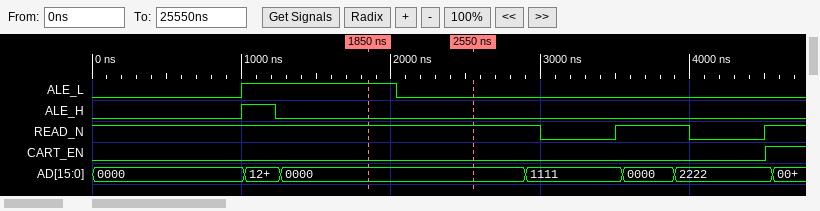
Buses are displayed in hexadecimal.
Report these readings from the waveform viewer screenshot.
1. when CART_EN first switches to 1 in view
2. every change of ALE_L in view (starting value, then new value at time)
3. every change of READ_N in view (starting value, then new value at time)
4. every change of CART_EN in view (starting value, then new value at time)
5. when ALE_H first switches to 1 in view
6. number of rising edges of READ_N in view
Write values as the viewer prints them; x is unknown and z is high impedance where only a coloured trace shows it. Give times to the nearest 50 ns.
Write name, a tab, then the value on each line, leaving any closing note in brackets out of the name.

when CART_EN first switches to 1 in view	4500 ns
every change of ALE_L in view	0, 1 at 1000 ns, 0 at 2050 ns
every change of READ_N in view	1, 0 at 3000 ns, 1 at 3500 ns, 0 at 4000 ns, 1 at 4500 ns
every change of CART_EN in view	0, 1 at 4500 ns
when ALE_H first switches to 1 in view	1000 ns
number of rising edges of READ_N in view	2
